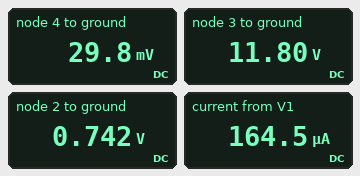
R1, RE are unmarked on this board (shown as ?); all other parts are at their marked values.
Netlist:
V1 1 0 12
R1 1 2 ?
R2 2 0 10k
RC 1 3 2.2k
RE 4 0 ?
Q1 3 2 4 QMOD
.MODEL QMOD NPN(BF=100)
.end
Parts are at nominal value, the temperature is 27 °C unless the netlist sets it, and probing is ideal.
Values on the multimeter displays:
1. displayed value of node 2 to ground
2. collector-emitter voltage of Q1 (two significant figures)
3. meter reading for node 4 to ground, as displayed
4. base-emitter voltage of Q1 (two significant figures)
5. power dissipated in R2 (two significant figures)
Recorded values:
0.742 V
12 V
29.8 mV
710 mV
55 µW
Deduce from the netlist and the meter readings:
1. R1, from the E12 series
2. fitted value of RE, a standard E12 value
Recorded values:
150 kΩ
330 Ω
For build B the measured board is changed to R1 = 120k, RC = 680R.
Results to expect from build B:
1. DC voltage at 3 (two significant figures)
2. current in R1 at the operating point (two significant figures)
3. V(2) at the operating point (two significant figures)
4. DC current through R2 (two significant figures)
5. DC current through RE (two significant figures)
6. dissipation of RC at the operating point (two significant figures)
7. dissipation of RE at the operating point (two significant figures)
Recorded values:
12 V
93 µA
890 mV
89 µA
410 µA
110 µW
55 µW
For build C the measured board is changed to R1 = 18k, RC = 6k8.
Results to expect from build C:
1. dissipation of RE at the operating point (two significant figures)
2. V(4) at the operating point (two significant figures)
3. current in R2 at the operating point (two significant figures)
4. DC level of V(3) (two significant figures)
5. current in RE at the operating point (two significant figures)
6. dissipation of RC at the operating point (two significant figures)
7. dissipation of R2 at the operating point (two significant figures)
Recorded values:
1.4 mW
690 mV
150 µA
740 mV
2.1 mA
19 mW
220 µW
